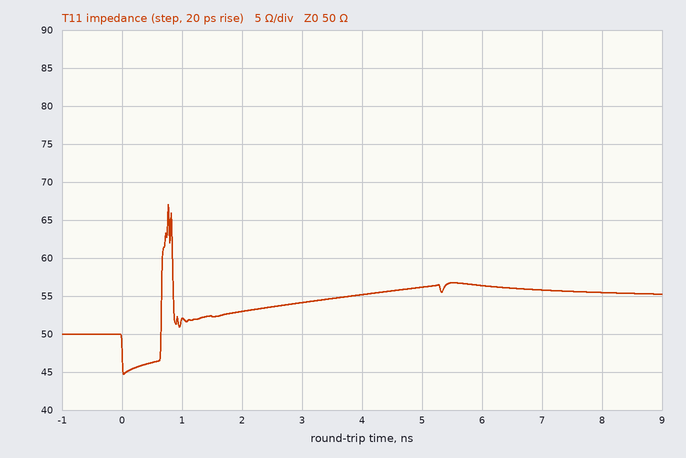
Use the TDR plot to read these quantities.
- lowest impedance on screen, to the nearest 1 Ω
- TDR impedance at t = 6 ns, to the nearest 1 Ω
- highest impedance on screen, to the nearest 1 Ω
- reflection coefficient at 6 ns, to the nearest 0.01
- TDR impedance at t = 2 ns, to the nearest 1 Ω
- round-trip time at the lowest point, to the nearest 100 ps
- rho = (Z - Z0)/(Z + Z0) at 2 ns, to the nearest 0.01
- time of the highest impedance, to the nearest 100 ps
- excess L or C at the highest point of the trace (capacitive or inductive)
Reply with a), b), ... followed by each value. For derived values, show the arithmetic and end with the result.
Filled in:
a) 45 Ω
b) 56 Ω
c) 67 Ω
d) (56 − 50)/(56 + 50) ≈ +0.06
e) 53 Ω
f) 0.0 ns
g) (53 − 50)/(53 + 50) ≈ +0.03
h) 800 ps
i) inductive
